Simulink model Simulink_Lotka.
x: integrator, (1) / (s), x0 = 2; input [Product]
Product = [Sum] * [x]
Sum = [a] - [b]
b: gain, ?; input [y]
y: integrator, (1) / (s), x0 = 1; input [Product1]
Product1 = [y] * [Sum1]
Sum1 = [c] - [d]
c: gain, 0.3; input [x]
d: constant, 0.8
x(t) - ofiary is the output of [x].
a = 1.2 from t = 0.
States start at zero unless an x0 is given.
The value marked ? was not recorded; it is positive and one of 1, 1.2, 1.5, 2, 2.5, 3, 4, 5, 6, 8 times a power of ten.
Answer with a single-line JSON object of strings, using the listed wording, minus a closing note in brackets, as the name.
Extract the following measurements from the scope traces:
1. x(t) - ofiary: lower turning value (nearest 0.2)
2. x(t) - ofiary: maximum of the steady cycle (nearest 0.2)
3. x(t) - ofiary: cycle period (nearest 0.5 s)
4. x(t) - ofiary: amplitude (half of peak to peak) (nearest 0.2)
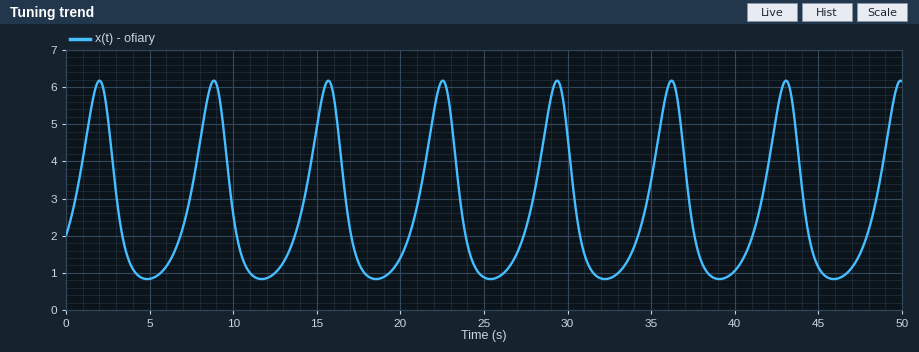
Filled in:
{"x(t) - ofiary: lower turning value": "0.8", "x(t) - ofiary: maximum of the steady cycle": "6.2", "x(t) - ofiary: cycle period": "7.0 s", "x(t) - ofiary: amplitude (half of peak to peak)": "2.6"}
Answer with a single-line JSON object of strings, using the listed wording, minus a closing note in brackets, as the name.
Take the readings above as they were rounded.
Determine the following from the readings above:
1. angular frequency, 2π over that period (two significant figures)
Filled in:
{"angular frequency, 2π over that period": "0.90 rad/s"}
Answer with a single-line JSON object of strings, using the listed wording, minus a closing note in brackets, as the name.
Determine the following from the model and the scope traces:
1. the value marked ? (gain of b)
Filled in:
{"the value marked ?": "0.5"}
